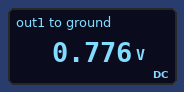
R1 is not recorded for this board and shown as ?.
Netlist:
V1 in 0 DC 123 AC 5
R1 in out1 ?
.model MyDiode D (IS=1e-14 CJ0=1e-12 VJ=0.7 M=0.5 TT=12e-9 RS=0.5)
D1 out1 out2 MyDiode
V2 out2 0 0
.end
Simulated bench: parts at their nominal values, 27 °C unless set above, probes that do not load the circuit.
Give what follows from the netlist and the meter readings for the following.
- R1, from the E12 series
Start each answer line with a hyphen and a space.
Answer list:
- 2.7 kΩ
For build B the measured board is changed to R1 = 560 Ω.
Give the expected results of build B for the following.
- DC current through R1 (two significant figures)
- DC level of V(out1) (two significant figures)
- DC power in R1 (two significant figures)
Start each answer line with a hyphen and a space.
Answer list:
- 220 mA
- 900 mV
- 27 W
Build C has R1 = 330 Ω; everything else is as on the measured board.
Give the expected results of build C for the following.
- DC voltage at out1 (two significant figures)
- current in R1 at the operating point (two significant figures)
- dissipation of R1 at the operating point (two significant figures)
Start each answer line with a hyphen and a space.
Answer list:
- 990 mV
- 370 mA
- 45 W
